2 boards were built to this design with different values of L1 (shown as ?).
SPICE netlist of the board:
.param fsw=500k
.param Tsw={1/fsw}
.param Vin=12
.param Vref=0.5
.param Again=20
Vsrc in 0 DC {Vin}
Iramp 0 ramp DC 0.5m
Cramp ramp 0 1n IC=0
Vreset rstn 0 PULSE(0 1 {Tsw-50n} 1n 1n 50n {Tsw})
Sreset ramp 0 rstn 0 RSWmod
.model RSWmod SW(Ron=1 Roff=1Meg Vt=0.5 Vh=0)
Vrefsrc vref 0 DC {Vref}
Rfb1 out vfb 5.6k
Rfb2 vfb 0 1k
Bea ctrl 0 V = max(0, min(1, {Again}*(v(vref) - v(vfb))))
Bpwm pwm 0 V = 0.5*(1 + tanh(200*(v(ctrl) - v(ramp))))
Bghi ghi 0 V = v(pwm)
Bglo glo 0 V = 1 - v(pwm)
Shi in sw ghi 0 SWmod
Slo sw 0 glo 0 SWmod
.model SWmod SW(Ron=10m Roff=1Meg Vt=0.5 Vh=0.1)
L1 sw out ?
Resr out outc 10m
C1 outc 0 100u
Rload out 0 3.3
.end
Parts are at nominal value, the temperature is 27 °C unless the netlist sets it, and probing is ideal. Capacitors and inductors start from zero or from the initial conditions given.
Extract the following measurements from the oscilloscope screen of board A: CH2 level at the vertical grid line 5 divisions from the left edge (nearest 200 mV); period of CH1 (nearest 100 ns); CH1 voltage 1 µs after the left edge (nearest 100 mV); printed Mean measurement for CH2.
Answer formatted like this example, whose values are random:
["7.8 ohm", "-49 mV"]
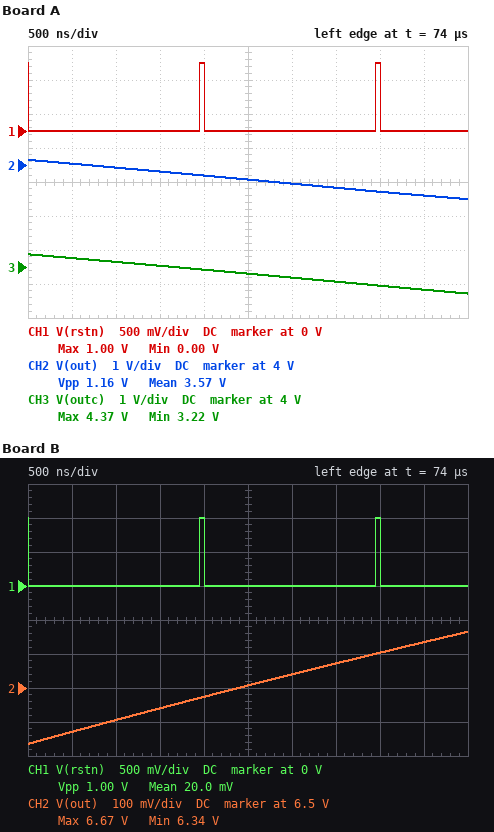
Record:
["3.6 V", "2.0 µs", "0 V", "3.57 V"]
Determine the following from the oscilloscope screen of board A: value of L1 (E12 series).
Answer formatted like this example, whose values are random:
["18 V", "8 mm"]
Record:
["6.8 µH"]
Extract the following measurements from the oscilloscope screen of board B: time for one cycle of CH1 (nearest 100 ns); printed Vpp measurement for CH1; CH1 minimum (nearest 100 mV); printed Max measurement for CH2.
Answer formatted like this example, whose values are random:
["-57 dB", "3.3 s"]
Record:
["2.0 µs", "1.00 V", "0 V", "6.67 V"]
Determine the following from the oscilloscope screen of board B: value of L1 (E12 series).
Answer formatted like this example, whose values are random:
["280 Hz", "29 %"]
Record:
["33 µH"]
